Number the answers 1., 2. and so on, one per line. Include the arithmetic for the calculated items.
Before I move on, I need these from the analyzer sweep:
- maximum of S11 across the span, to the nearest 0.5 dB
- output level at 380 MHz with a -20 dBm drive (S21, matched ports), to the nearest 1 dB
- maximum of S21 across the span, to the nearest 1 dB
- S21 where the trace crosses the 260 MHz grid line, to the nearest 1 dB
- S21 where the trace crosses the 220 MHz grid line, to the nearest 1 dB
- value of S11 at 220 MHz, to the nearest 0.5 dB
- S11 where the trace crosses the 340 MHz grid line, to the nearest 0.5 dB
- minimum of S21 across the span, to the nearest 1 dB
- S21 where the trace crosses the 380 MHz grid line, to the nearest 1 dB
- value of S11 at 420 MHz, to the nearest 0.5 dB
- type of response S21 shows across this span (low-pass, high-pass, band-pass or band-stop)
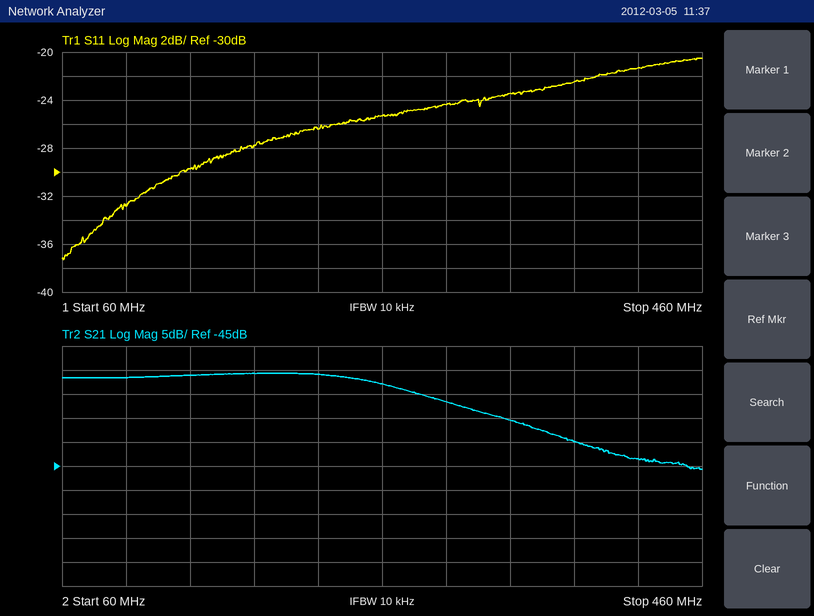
1. -20.5 dB
2. -20 dBm + (-40 dB) = -60 dBm
3. -26 dB
4. -28 dB
5. -26 dB
6. -26.5 dB
7. -23.5 dB
8. -46 dB
9. -40 dB
10. -21.5 dB
11. low-pass
